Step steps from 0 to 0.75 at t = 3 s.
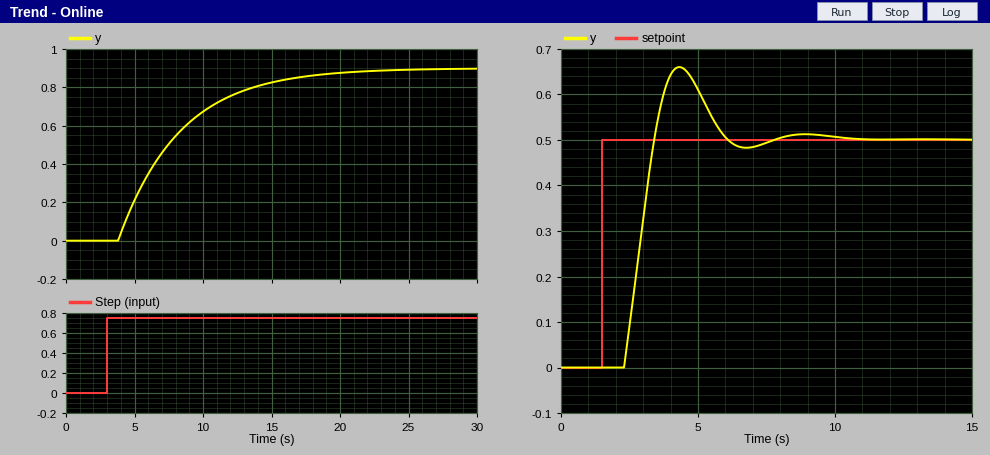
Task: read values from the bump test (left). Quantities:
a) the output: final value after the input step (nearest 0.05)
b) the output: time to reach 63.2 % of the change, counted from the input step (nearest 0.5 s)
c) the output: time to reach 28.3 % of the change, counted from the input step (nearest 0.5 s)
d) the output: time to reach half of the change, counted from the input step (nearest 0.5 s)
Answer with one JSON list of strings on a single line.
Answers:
["0.90", "5.5 s", "2.5 s", "4.0 s"]
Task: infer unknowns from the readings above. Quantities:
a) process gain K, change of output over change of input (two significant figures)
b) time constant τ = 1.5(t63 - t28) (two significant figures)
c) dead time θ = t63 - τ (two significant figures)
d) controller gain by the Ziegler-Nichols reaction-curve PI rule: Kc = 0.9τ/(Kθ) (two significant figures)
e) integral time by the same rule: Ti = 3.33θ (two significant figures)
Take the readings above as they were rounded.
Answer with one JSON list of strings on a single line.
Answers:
["1.2", "4.5 s", "1.0 s", "3.4", "3.3 s"]
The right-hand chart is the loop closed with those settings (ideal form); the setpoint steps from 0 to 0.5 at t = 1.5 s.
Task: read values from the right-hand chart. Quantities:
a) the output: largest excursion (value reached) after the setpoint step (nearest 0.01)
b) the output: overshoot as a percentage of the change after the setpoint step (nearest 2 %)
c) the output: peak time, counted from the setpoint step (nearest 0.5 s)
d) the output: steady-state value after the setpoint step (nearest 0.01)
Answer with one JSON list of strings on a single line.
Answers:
["0.66", "32 %", "3.0 s", "0.50"]
